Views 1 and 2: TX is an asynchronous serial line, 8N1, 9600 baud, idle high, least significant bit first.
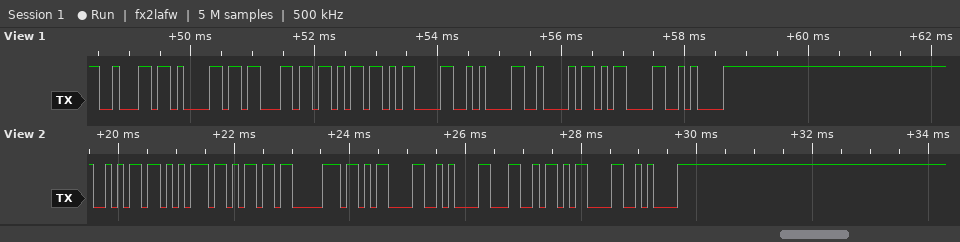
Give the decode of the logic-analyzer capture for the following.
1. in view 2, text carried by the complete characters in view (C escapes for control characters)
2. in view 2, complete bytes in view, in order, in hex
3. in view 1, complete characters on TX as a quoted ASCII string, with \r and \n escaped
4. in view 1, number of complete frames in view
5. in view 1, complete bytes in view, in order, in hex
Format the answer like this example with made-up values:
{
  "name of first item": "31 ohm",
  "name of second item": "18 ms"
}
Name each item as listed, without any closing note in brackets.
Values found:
{
  "in view 2, text carried by the complete characters in view": "\"jump\\r\\nL\\r\\n\"",
  "in view 2, complete bytes in view, in order, in hex": "6A 75 6D 70 0D 0A 4C 0D 0A",
  "in view 1, complete characters on TX as a quoted ASCII string, with \\r and \\n escaped": "\"back\\r\\nB\\r\\n\"",
  "in view 1, number of complete frames in view": "9",
  "in view 1, complete bytes in view, in order, in hex": "62 61 63 6B 0D 0A 42 0D 0A"
}
